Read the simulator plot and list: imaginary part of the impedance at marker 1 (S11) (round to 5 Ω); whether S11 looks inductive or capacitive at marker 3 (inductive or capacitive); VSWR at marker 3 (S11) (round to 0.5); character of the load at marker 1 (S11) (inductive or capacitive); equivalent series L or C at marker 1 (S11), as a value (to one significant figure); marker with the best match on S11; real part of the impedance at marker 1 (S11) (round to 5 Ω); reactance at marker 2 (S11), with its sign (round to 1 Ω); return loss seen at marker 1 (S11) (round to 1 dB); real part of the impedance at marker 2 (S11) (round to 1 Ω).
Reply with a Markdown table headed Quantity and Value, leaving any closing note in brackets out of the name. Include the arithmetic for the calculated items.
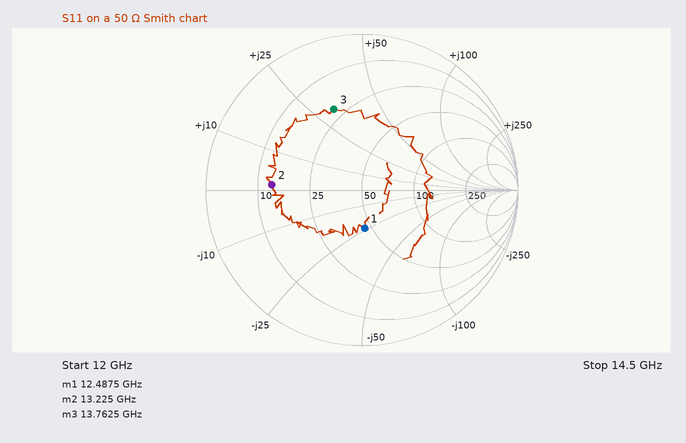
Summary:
| Quantity | Value |
|---|---|
| imaginary part of the impedance at marker 1 (S11) | -25 Ω |
| whether S11 looks inductive or capacitive at marker 3 | inductive |
| VSWR at marker 3 (S11) | 3.5 |
| character of the load at marker 1 (S11) | capacitive |
| equivalent series L or C at marker 1 (S11), as a value | C = 1/(2π × 12.4875 GHz × 25 Ω) ≈ 510 fF, so 500 fF to one significant figure |
| marker with the best match on S11 | marker 1 |
| real part of the impedance at marker 1 (S11) | 45 Ω |
| reactance at marker 2 (S11), with its sign | +1 Ω |
| return loss seen at marker 1 (S11) | 12 dB |
| real part of the impedance at marker 2 (S11) | 13 Ω |
